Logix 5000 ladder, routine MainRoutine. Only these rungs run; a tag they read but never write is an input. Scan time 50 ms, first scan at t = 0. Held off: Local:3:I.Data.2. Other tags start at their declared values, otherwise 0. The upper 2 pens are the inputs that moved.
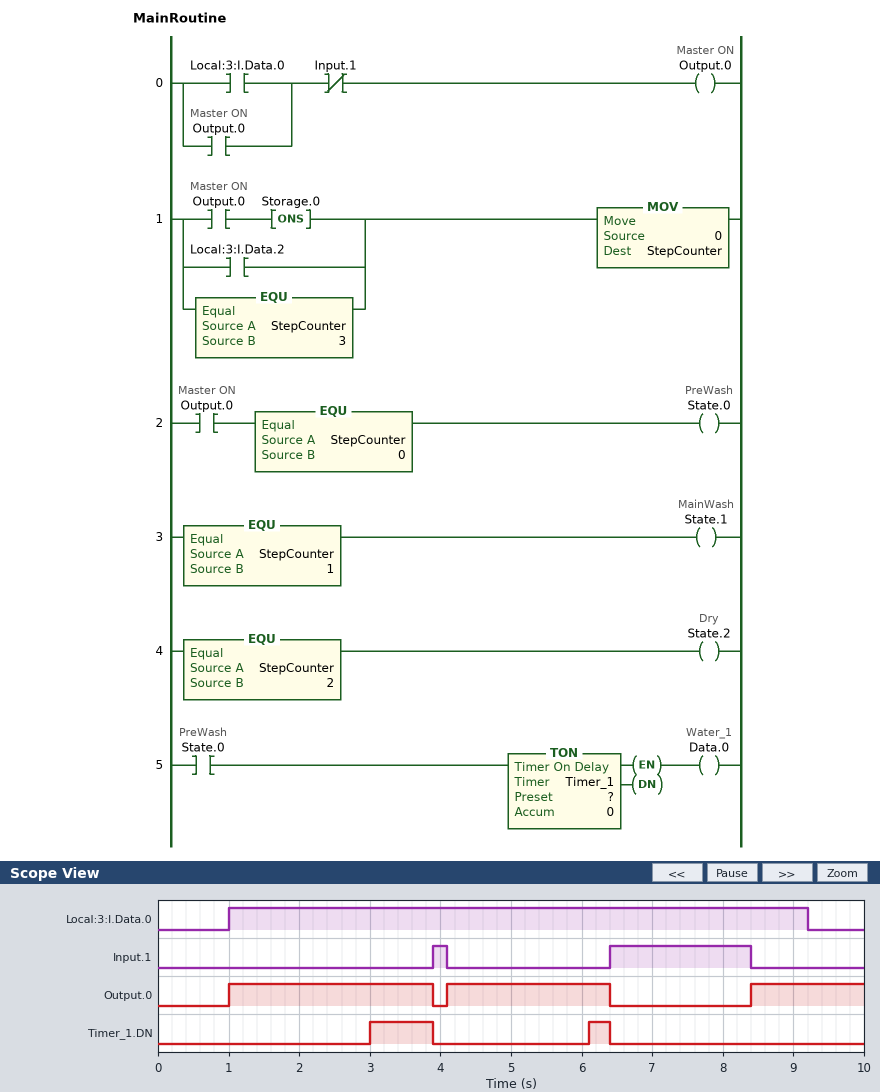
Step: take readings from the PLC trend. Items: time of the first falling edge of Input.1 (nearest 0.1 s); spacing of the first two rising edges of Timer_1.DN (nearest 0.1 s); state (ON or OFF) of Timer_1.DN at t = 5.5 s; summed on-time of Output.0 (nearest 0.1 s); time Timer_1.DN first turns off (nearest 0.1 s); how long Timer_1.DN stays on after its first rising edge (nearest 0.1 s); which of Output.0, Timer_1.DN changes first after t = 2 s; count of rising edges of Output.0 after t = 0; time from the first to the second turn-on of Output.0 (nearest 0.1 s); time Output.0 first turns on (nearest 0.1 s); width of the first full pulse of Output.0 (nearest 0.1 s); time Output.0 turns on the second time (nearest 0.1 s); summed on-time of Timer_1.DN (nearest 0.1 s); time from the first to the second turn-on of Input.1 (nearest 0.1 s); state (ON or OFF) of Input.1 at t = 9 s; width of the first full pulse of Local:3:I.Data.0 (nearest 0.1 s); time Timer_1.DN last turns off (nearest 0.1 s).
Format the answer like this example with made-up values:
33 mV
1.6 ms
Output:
4.1 s
3.1 s
OFF
6.8 s
3.9 s
0.9 s
Timer_1.DN
3
3.1 s
1.0 s
2.9 s
4.1 s
1.2 s
2.5 s
OFF
8.2 s
6.4 s
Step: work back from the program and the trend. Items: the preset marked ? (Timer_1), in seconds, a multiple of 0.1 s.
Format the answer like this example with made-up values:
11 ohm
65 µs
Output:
2.0 s
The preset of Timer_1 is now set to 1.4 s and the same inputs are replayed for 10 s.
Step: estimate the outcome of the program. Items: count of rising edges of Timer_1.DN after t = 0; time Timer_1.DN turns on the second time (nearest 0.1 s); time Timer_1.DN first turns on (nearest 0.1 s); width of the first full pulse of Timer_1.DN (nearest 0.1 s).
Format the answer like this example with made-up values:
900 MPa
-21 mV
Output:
3
5.5 s
2.4 s
1.5 s
